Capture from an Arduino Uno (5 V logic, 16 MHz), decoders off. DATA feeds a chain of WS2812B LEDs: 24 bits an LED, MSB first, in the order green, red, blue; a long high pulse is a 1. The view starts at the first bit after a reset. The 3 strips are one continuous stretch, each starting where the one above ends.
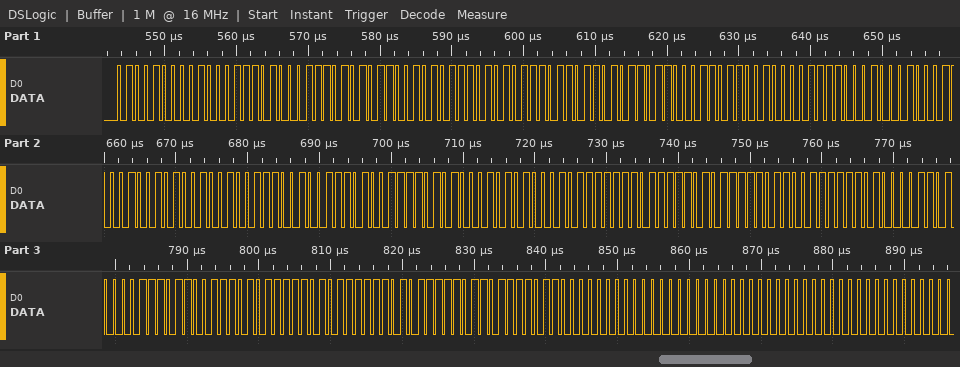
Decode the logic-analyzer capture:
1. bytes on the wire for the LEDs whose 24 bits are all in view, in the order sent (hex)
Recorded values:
48 47 47 56 57 57 6D 6C 6C 87 88 88 94 93 93 A7 A8 A8 BF BE BE CF D0 D0 EC EB EB F5 F6 F6 00 00 00
